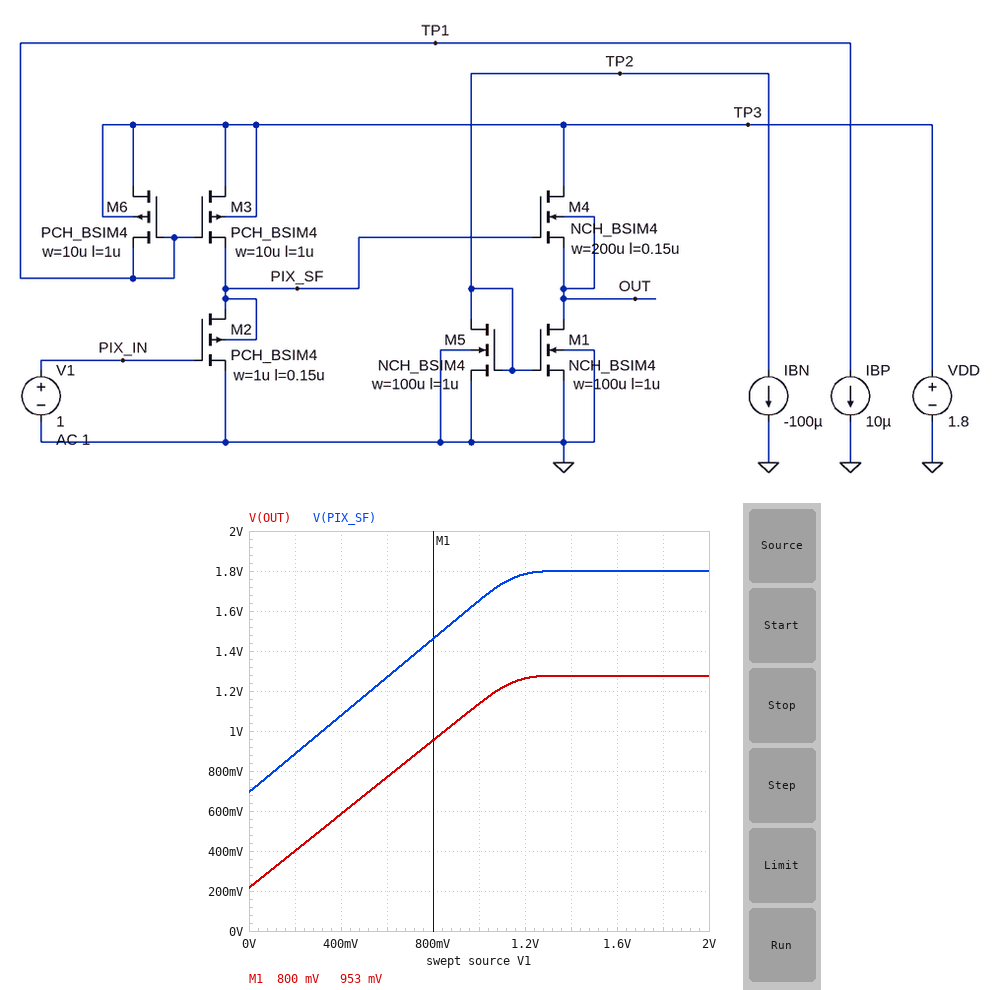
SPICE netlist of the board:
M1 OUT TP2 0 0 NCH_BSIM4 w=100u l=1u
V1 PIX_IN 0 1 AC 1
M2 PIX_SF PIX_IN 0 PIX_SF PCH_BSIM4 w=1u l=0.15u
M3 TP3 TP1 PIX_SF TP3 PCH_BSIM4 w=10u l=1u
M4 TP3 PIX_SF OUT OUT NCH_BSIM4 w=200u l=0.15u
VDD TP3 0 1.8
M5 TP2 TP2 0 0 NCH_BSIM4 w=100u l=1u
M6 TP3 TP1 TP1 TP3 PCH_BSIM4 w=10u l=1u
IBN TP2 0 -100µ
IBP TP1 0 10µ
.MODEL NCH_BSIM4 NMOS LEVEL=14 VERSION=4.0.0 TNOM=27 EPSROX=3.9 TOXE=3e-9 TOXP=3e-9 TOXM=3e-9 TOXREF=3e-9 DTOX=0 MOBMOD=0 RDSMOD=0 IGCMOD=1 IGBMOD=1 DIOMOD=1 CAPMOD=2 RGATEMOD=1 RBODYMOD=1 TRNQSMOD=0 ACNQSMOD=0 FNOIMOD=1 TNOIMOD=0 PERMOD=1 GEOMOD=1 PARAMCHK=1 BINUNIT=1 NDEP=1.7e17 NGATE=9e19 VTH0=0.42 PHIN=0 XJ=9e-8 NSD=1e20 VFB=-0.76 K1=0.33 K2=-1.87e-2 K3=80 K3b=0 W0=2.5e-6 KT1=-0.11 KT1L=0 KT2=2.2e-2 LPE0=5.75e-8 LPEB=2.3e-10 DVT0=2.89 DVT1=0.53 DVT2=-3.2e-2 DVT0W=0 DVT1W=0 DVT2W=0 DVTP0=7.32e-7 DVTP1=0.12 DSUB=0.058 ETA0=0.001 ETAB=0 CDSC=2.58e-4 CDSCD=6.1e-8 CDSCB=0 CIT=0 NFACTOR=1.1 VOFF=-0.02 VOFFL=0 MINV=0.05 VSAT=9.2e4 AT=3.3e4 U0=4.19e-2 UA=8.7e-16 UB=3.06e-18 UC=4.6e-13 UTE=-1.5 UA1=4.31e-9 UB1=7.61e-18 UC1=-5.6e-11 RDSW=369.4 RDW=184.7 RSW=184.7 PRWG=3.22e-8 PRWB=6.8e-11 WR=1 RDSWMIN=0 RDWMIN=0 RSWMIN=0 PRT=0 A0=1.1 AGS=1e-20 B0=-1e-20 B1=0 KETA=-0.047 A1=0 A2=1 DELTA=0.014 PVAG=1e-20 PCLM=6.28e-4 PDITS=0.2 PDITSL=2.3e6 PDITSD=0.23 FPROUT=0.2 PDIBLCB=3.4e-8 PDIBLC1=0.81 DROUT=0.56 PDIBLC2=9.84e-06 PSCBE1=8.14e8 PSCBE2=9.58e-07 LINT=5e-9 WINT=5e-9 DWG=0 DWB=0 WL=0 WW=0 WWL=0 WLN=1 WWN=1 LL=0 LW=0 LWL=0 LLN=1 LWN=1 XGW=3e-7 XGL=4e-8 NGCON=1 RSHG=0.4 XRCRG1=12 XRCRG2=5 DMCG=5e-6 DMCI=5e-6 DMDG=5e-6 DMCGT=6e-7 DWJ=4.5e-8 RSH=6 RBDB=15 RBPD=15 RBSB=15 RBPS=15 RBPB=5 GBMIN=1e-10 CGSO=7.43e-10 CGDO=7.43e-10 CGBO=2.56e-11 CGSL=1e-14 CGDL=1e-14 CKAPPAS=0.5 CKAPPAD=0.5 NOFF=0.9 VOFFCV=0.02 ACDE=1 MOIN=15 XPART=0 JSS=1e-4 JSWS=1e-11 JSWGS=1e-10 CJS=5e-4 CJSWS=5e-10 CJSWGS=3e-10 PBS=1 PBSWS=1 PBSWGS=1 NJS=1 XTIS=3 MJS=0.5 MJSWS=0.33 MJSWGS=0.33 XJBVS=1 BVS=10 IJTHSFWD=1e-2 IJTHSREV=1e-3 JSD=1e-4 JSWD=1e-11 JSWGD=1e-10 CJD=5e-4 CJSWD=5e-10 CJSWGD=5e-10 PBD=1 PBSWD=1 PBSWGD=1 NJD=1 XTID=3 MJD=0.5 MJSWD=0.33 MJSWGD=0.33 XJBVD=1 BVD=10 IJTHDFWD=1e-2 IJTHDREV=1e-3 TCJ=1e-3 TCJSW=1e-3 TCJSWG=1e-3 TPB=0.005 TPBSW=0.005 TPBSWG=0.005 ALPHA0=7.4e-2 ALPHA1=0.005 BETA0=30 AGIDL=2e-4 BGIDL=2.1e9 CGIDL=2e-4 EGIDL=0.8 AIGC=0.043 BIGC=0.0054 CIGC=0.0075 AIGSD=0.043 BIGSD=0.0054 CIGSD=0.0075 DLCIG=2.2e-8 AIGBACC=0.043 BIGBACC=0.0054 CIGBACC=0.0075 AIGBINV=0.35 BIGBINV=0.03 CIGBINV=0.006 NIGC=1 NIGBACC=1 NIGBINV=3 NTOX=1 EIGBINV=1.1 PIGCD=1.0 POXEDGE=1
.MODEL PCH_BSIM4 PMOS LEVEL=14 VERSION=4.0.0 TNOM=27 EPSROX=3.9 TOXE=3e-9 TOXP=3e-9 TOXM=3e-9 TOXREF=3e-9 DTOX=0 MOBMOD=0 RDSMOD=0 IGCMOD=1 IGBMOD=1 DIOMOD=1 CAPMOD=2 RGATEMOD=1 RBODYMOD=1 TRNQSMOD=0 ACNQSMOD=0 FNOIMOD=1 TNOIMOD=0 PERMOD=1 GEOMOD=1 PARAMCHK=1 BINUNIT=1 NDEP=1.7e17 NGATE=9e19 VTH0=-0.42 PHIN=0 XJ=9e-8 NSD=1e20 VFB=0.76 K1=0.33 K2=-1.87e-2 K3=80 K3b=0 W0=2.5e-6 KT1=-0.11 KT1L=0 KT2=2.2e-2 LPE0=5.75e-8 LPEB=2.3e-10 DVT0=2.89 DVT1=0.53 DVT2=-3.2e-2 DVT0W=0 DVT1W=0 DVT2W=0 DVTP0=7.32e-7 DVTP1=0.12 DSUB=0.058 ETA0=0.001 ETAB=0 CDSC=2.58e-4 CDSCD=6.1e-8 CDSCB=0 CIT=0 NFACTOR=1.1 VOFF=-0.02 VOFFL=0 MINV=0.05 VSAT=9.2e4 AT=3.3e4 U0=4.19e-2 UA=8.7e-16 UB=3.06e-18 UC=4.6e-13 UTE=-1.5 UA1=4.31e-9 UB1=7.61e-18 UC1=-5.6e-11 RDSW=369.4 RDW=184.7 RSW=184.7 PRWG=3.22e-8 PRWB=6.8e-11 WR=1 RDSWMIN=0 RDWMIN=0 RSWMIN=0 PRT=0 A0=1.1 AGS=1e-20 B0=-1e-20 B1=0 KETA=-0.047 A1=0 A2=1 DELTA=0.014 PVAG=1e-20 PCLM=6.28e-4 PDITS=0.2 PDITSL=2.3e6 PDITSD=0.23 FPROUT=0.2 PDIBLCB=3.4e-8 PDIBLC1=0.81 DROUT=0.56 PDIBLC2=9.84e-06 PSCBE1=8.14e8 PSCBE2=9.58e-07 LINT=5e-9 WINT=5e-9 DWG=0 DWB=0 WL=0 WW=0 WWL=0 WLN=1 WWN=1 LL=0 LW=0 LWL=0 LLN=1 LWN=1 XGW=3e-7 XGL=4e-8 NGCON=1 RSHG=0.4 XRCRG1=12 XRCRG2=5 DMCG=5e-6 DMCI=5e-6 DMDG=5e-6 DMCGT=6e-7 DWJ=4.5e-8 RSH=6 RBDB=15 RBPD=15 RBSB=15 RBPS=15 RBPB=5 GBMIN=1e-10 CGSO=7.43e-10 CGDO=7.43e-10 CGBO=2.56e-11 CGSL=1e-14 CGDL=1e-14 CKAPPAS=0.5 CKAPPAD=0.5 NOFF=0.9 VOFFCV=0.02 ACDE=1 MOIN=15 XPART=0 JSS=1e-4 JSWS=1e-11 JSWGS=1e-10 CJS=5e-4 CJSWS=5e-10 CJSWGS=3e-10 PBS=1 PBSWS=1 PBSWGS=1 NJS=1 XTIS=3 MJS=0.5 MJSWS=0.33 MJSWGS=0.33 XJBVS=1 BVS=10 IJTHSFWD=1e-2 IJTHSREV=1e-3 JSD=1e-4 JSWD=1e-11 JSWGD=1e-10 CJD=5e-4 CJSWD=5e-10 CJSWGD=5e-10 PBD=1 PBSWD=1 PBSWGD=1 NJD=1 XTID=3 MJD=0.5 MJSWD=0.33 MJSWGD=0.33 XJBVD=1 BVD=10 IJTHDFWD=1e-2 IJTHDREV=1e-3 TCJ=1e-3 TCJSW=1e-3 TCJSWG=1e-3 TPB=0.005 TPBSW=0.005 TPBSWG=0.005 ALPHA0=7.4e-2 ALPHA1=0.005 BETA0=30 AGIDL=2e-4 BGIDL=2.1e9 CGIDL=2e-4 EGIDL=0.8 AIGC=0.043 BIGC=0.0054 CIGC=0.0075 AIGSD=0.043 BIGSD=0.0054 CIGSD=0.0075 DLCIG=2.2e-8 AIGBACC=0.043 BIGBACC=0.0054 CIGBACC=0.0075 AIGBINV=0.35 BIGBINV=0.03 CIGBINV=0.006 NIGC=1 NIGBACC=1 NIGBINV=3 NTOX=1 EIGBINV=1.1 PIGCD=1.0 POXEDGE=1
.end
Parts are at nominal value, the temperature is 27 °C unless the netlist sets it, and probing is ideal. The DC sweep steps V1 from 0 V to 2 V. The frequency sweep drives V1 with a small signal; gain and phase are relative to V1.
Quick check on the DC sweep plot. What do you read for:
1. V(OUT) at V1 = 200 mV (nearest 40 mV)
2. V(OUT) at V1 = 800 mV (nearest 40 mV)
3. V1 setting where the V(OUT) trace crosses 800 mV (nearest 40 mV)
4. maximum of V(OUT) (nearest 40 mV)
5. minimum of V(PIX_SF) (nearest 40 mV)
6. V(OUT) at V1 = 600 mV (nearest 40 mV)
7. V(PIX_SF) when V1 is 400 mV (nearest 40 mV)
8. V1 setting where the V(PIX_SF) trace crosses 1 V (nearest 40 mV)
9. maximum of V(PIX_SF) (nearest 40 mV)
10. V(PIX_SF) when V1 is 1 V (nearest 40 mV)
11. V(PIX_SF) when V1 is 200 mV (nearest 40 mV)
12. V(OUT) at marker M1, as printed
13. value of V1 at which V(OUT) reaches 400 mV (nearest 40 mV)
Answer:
400 mV
960 mV
640 mV
1.28 V
680 mV
760 mV
1.08 V
320 mV
1.80 V
1.64 V
880 mV
953 mV
200 mV
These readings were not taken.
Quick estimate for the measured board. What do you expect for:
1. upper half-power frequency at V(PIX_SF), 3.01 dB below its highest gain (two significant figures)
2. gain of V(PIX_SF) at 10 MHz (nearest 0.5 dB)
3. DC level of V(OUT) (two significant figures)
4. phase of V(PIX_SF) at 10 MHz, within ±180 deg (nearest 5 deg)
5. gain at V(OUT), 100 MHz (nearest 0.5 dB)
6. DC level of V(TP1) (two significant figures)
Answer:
120 MHz
-0.5 dB
1.1 V
-5 deg
-3.5 dB
1.2 V
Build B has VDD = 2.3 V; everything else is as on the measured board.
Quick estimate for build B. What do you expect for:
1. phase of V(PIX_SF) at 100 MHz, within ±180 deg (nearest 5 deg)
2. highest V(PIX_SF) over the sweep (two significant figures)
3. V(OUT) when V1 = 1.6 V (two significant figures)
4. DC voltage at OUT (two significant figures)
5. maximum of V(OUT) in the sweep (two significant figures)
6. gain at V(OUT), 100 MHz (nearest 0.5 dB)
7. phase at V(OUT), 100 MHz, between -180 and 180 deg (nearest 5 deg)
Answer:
-40 deg
2.3 V
1.7 V
1.2 V
1.8 V
-3.0 dB
-50 deg
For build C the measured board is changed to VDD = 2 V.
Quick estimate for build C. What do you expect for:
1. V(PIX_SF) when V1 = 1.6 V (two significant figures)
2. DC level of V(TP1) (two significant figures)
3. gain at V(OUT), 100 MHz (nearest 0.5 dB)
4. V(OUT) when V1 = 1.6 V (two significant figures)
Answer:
2.0 V
1.4 V
-3.0 dB
1.5 V
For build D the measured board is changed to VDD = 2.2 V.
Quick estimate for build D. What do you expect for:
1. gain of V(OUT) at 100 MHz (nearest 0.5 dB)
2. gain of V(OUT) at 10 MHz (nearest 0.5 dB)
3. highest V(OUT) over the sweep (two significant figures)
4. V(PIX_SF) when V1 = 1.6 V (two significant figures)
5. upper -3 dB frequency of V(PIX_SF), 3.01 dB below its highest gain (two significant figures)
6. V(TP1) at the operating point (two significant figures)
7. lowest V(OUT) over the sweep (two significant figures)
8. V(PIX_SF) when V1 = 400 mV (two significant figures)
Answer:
-3.0 dB
-0.5 dB
1.7 V
2.2 V
130 MHz
1.6 V
230 mV
1.1 V
